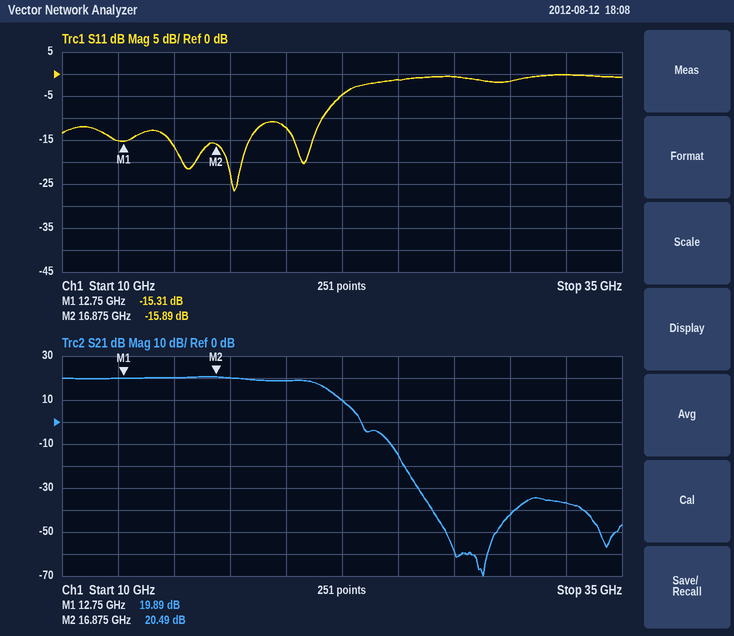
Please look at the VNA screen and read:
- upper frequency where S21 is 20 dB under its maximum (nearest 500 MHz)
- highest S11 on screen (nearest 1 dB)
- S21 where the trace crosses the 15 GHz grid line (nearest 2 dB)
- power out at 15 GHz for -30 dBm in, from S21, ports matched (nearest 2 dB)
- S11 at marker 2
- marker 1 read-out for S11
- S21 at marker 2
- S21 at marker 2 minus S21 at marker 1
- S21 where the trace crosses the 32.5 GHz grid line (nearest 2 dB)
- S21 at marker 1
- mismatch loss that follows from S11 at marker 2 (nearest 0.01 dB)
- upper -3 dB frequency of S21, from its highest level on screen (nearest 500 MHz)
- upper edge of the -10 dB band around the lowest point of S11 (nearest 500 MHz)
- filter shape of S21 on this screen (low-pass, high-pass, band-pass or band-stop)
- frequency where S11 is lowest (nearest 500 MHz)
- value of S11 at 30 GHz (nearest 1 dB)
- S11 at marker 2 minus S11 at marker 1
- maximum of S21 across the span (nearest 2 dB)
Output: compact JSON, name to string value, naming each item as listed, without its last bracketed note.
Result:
{"upper frequency where S21 is 20 dB under its maximum": "23.5 GHz", "highest S11 on screen": "0 dB", "S21 where the trace crosses the 15 GHz grid line": "20 dB", "power out at 15 GHz for -30 dBm in, from S21, ports matched": "-10 dBm", "S11 at marker 2": "-15.89 dB", "marker 1 read-out for S11": "-15.31 dB", "S21 at marker 2": "20.49 dB", "S21 at marker 2 minus S21 at marker 1": "0.60 dB", "S21 where the trace crosses the 32.5 GHz grid line": "-36 dB", "S21 at marker 1": "19.89 dB", "mismatch loss that follows from S11 at marker 2": "0.11 dB", "upper -3 dB frequency of S21, from its highest level on screen": "21.5 GHz", "upper edge of the -10 dB band around the lowest point of S11": "21.5 GHz", "filter shape of S21 on this screen": "low-pass", "frequency where S11 is lowest": "17.5 GHz", "value of S11 at 30 GHz": "-2 dB", "S11 at marker 2 minus S11 at marker 1": "-0.58 dB", "maximum of S21 across the span": "20 dB"}
